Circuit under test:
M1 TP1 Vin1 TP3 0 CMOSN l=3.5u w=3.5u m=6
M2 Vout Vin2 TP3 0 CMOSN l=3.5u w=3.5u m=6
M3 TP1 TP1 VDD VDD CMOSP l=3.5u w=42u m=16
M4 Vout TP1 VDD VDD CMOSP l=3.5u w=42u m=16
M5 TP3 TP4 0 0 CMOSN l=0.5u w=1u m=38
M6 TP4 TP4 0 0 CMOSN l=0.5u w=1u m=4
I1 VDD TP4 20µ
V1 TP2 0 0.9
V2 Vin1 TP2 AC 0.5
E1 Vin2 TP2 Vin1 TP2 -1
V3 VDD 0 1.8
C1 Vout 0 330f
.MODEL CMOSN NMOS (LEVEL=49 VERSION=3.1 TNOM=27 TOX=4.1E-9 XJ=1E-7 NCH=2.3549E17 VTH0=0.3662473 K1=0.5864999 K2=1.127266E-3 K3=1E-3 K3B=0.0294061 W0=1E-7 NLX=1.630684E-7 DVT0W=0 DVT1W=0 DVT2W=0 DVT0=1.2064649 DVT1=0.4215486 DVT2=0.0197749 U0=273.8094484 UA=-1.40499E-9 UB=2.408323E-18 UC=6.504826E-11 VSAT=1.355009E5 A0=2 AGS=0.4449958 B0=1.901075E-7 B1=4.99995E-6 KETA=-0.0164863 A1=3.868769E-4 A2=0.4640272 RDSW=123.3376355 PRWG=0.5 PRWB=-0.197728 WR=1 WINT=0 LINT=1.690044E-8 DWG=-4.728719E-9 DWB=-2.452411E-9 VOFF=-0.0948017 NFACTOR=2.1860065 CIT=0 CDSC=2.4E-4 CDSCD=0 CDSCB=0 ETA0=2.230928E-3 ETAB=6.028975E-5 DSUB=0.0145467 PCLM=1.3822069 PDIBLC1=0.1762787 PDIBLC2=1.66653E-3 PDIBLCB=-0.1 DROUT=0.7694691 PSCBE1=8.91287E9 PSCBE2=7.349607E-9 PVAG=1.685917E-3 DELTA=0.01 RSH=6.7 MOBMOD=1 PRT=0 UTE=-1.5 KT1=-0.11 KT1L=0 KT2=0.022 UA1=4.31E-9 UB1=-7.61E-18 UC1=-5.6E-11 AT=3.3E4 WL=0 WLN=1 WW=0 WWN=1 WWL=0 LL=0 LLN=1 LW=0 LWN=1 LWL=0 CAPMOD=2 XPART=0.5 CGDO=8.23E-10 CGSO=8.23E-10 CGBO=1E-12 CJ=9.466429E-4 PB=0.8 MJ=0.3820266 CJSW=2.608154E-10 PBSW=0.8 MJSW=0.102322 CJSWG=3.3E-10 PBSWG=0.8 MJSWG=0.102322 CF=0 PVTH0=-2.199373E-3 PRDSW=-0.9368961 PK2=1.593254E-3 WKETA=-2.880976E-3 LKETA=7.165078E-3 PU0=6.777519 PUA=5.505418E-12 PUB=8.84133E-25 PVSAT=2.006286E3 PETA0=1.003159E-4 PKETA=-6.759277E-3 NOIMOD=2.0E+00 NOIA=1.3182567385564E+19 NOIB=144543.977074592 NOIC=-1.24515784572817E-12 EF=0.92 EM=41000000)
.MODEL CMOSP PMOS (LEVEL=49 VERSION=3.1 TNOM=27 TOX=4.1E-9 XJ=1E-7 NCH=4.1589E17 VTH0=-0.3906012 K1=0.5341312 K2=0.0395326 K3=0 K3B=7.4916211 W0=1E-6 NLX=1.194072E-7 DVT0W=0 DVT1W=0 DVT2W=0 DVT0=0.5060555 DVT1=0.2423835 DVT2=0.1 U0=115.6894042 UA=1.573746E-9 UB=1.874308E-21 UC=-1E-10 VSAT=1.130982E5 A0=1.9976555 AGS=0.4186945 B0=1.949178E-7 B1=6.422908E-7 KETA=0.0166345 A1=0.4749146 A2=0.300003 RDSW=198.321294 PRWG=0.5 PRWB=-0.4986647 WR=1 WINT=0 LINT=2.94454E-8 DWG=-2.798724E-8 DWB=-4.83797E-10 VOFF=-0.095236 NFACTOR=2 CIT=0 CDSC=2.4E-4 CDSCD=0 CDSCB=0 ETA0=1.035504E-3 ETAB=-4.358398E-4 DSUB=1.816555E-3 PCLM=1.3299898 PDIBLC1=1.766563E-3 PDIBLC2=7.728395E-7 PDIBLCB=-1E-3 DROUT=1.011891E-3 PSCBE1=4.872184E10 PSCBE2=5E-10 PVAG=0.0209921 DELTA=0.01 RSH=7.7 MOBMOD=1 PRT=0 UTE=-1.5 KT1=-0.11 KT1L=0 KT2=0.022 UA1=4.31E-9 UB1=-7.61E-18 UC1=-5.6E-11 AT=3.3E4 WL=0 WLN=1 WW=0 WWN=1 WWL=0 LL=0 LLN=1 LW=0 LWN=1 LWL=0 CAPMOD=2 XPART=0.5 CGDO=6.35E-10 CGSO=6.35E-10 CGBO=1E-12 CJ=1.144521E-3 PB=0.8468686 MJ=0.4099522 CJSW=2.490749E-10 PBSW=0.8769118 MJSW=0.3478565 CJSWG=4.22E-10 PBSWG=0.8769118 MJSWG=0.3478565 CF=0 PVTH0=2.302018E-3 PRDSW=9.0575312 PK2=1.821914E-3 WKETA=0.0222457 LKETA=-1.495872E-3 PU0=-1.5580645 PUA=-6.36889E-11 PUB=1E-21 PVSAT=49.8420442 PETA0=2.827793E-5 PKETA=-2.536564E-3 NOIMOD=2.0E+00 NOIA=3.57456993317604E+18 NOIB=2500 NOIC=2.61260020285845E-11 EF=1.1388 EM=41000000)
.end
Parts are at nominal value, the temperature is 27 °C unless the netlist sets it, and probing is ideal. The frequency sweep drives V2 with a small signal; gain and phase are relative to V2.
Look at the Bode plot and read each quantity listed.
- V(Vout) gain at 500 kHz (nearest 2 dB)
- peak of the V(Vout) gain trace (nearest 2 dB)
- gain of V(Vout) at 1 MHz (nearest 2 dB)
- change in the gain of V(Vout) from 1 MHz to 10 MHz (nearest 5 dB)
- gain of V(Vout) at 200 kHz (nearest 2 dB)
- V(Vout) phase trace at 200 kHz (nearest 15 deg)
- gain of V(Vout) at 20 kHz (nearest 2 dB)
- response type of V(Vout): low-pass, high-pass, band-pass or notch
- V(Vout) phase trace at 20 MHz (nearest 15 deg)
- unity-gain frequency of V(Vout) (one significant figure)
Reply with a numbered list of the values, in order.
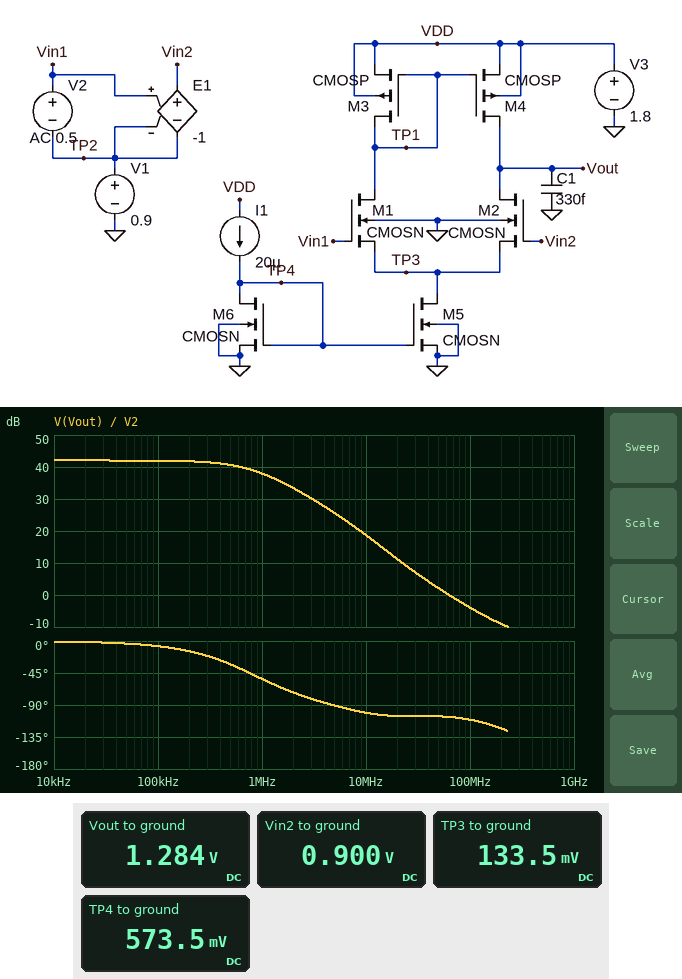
1. 40 dB
2. 42 dB
3. 38 dB
4. -20 dB
5. 42 dB
6. -15 deg
7. 42 dB
8. low-pass
9. -105 deg
10. 60 MHz
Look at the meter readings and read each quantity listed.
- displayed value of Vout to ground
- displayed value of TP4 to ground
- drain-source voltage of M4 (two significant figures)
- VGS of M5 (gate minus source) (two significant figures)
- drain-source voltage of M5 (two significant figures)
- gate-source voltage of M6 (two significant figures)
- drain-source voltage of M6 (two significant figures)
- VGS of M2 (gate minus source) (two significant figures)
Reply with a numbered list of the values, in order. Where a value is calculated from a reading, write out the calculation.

1. 1.284 V
2. 573.5 mV
3. 1.284 V - 1.8 V = -520 mV
4. 573.5 mV = 570 mV
5. 133.5 mV = 130 mV
6. 573.5 mV = 570 mV
7. 573.5 mV = 570 mV
8. 900 mV - 133.5 mV = 770 mV
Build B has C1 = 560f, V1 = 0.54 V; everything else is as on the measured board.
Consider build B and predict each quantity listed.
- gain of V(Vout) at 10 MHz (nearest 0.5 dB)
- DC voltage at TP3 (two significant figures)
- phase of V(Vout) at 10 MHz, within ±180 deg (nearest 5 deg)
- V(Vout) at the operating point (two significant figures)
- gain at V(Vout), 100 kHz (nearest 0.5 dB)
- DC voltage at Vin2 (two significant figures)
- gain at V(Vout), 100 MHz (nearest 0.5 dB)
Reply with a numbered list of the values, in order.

1. 7.0 dB
2. 12 mV
3. -105 deg
4. 1.4 V
5. 44.5 dB
6. 540 mV
7. -12.0 dB
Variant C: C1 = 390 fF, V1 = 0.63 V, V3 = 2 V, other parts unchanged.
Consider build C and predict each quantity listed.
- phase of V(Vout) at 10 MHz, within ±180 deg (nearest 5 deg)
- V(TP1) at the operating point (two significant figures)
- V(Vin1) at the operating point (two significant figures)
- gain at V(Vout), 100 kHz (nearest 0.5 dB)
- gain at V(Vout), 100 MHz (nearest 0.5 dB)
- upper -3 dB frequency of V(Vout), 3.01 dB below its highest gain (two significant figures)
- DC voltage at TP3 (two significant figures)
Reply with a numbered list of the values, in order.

1. -105 deg
2. 1.5 V
3. 630 mV
4. 44.0 dB
5. -8.0 dB
6. 380 kHz
7. 27 mV
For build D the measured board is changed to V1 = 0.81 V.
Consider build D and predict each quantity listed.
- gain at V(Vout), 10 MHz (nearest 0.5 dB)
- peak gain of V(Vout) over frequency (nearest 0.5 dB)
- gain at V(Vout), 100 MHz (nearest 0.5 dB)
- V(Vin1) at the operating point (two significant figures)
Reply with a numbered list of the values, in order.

1. 18.0 dB
2. 42.5 dB
3. -4.5 dB
4. 810 mV
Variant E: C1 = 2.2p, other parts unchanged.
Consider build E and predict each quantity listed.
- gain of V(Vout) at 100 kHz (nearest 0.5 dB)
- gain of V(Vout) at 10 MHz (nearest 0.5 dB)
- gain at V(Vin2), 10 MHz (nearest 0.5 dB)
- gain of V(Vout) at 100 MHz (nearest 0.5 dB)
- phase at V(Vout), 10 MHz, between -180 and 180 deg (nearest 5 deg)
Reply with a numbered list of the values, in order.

1. 41.5 dB
2. 10.5 dB
3. 0 dB
4. -13.5 dB
5. -110 deg
